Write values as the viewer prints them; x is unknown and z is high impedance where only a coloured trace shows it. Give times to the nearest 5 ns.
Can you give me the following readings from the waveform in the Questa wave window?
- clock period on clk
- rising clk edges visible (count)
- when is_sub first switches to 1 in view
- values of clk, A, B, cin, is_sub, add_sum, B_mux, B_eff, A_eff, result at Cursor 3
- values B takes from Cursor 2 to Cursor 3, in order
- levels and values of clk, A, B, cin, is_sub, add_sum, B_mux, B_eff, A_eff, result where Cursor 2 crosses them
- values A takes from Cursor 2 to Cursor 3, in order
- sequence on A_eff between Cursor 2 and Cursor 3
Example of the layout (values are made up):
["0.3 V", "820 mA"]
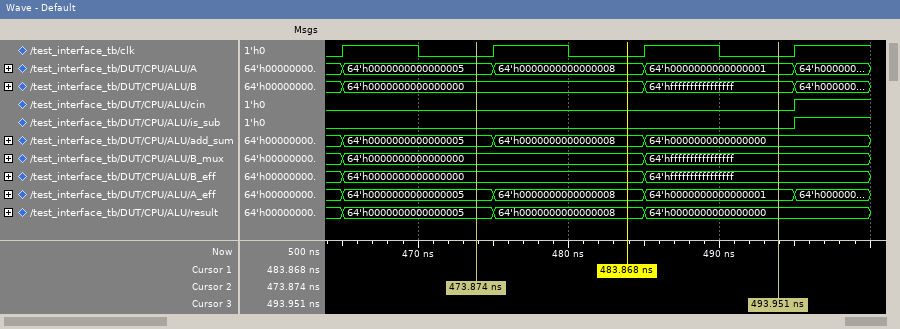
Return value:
["10 ns", "4", "495 ns", "clk=0, A=64'h0000000000000001, B=64'hffffffffffffffff, cin=0, is_sub=0, add_sum=64'h0000000000000000, B_mux=64'hffffffffffffffff, B_eff=64'hffffffffffffffff, A_eff=64'h0000000000000001, result=64'h0000000000000000", "64'h0000000000000000, 64'hffffffffffffffff", "clk=0, A=64'h0000000000000005, B=64'h0000000000000000, cin=0, is_sub=0, add_sum=64'h0000000000000005, B_mux=64'h0000000000000000, B_eff=64'h0000000000000000, A_eff=64'h0000000000000005, result=64'h0000000000000005", "64'h0000000000000005, 64'h0000000000000008, 64'h0000000000000001", "64'h0000000000000005, 64'h0000000000000008, 64'h0000000000000001"]
